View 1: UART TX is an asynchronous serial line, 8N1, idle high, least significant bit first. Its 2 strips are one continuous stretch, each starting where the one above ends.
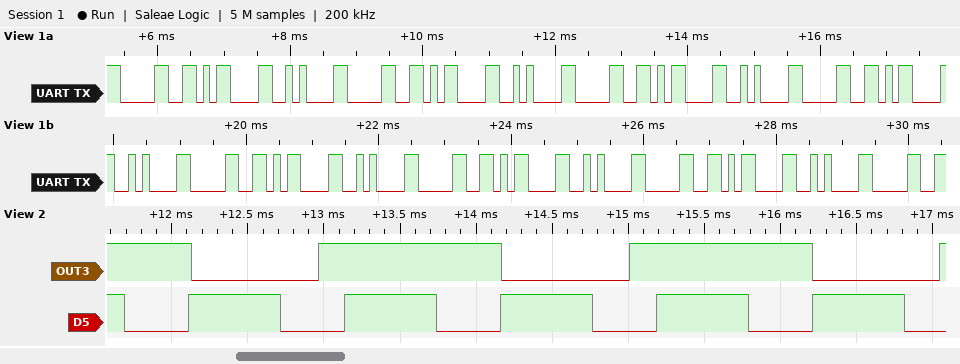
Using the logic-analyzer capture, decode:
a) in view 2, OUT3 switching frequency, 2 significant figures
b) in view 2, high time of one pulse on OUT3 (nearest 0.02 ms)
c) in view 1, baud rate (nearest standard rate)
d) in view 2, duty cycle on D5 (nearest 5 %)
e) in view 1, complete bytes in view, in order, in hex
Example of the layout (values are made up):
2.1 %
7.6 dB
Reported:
490 Hz
1.20 ms
9600 baud
60 %
0x30 0x0D 0x0A 0x30 0x0D 0x0A 0x30 0x0D 0x0A 0x30 0x0D 0x0A 0x30 0x0D 0x0A 0x30 0x0D 0x0A 0x30 0x0D 0x0A 0x30
